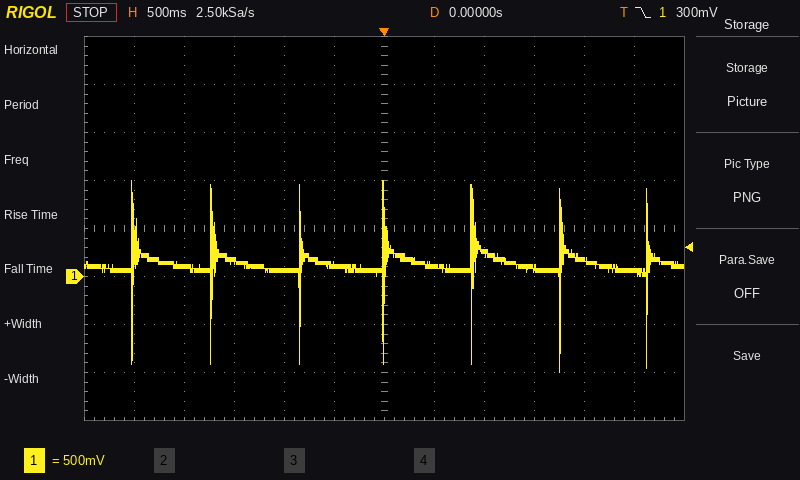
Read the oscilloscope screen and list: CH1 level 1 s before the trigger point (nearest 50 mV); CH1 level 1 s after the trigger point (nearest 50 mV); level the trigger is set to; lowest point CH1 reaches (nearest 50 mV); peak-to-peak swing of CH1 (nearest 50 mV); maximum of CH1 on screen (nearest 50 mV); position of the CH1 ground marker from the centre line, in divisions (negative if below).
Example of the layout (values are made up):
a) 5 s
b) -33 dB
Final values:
a) 50 mV
b) 250 mV
c) 300 mV
d) -1.00 V
e) 2.00 V
f) 1.00 V
g) -1.0 div
